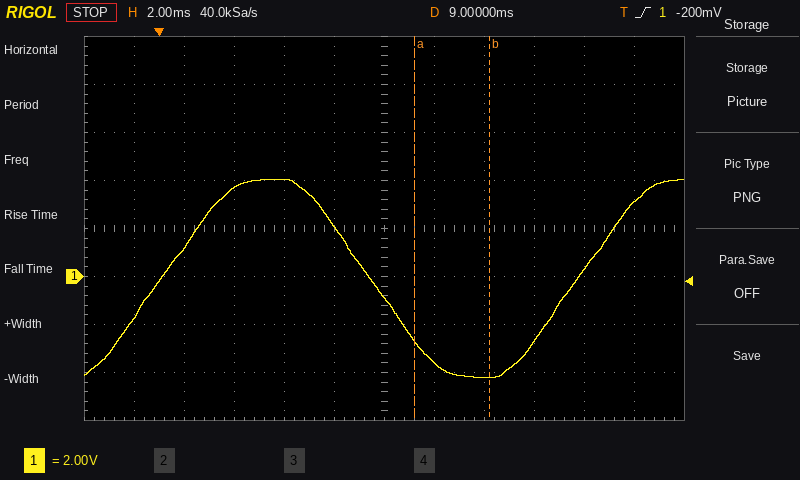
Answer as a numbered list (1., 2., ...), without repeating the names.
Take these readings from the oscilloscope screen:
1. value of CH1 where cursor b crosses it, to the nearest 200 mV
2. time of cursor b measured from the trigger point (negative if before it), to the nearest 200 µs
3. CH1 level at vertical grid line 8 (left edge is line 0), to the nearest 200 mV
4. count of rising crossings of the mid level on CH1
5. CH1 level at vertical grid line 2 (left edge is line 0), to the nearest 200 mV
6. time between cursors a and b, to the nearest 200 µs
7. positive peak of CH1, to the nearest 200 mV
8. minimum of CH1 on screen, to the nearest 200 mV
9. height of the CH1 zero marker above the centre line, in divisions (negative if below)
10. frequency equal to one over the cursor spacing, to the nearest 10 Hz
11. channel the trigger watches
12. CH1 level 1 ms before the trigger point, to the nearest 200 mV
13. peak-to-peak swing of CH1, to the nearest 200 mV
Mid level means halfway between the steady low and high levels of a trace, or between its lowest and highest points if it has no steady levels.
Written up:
1. -4.2 V
2. +13.2 ms
3. -4.2 V
4. 2
5. 1.2 V
6. 3.0 ms
7. 4.0 V
8. -4.2 V
9. -1.0 div
10. 330 Hz
11. CH1
12. -1.8 V
13. 8.2 V
